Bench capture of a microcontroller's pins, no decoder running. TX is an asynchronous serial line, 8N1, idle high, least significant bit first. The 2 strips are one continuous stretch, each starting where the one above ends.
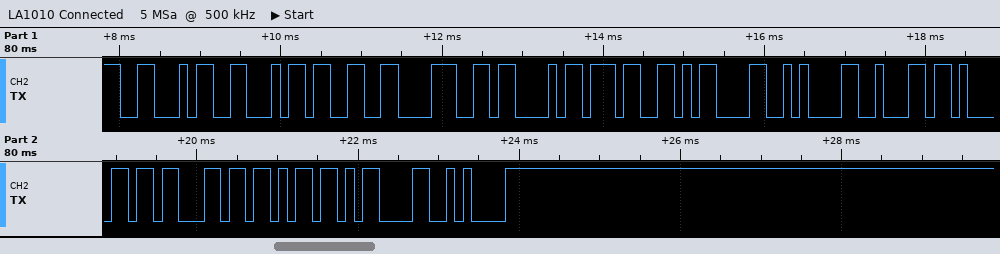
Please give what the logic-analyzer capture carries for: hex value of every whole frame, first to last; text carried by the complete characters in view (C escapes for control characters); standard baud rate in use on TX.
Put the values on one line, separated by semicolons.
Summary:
46 46 33 38 43 37 0D 0A 62 61 63 6B 0D 0A; "FF38C7\r\nback\r\n"; 9600 baud
